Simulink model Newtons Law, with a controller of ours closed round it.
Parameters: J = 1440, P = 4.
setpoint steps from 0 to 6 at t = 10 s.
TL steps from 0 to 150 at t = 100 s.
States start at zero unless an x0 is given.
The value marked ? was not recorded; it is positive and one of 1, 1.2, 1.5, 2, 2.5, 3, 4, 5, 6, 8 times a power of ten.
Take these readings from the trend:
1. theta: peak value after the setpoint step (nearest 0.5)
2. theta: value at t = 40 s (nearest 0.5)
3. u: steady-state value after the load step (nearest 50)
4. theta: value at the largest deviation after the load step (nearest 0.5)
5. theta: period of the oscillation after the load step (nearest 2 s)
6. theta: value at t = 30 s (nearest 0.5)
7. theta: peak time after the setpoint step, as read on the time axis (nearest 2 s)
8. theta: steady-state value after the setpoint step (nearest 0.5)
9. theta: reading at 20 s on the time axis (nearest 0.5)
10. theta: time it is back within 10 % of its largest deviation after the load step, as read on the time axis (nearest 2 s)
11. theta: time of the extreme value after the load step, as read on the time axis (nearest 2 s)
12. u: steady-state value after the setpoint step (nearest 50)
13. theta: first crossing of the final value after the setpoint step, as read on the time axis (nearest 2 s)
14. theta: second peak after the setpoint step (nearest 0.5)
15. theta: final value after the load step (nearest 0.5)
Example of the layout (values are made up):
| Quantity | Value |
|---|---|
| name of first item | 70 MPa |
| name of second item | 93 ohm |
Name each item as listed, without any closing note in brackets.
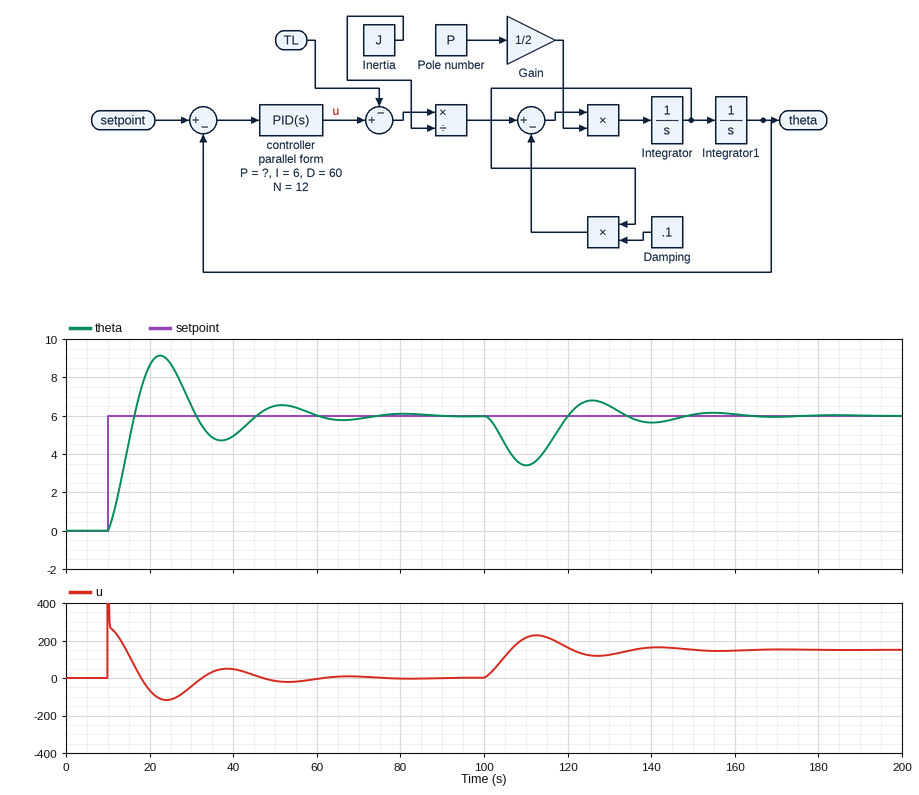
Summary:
| Quantity | Value |
|---|---|
| theta: peak value after the setpoint step | 9.0 |
| theta: value at t = 40 s | 5.0 |
| u: steady-state value after the load step | 150 |
| theta: value at the largest deviation after the load step | 3.5 |
| theta: period of the oscillation after the load step | 30 s |
| theta: value at t = 30 s | 6.5 |
| theta: peak time after the setpoint step, as read on the time axis | 22 s |
| theta: steady-state value after the setpoint step | 6.0 |
| theta: reading at 20 s on the time axis | 8.5 |
| theta: time it is back within 10 % of its largest deviation after the load step, as read on the time axis | 144 s |
| theta: time of the extreme value after the load step, as read on the time axis | 110 s |
| u: steady-state value after the setpoint step | 0 |
| theta: first crossing of the final value after the setpoint step, as read on the time axis | 16 s |
| theta: second peak after the setpoint step | 6.5 |
| theta: final value after the load step | 6.0 |
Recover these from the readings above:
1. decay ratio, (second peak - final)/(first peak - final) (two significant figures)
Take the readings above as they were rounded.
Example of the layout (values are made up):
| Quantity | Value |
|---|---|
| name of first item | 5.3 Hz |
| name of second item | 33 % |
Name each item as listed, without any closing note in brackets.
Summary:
| Quantity | Value |
|---|---|
| decay ratio, (second peak - final)/(first peak - final) | 0.17 |
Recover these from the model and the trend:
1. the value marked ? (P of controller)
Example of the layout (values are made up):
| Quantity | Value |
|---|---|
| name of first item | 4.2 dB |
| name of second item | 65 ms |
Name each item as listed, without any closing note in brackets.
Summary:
| Quantity | Value |
|---|---|
| the value marked ? | 50 |
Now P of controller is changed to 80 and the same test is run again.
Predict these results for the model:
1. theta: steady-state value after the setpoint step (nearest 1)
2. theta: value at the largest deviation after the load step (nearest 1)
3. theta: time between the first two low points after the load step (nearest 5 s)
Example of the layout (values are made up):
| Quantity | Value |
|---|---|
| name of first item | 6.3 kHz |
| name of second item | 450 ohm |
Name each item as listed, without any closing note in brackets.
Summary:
| Quantity | Value |
|---|---|
| theta: steady-state value after the setpoint step | 6 |
| theta: value at the largest deviation after the load step | 4 |
| theta: time between the first two low points after the load step | 20 s |
